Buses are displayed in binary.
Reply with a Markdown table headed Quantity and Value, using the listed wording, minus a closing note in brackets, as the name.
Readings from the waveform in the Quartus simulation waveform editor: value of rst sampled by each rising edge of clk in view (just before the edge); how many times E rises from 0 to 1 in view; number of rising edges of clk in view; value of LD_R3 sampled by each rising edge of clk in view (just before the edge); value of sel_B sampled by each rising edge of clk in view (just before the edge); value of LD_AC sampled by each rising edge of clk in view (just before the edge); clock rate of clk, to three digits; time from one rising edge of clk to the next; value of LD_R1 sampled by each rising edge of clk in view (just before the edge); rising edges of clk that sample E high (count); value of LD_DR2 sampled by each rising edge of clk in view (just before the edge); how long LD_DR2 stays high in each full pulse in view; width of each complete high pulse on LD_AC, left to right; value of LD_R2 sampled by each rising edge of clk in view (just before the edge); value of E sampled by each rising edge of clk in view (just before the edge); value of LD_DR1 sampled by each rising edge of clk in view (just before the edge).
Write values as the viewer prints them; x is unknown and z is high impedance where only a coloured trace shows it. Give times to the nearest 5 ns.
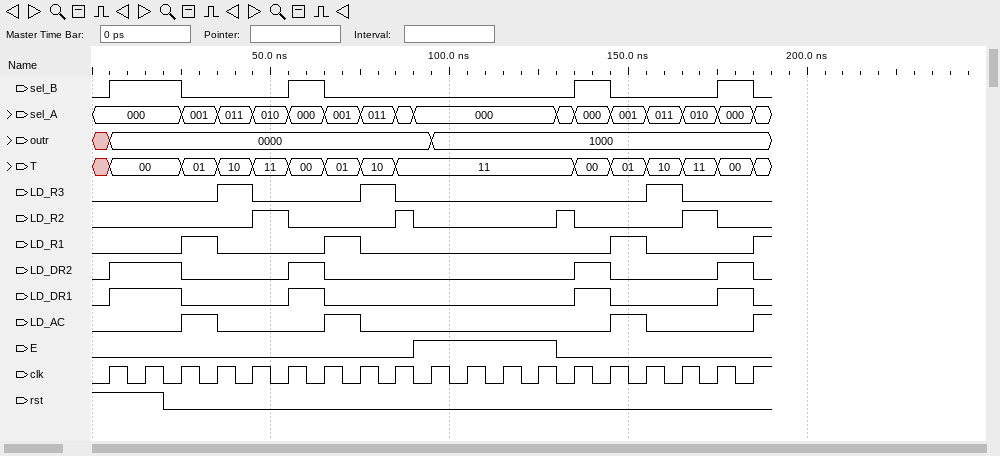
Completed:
| Quantity | Value |
|---|---|
| value of rst sampled by each rising edge of clk in view | 1 1 0 0 0 0 0 0 0 0 0 0 0 0 0 0 0 0 0 |
| how many times E rises from 0 to 1 in view | 1 |
| number of rising edges of clk in view | 19 |
| value of LD_R3 sampled by each rising edge of clk in view | 0 0 0 0 1 0 0 0 1 0 0 0 0 0 0 0 1 0 0 |
| value of sel_B sampled by each rising edge of clk in view | 0 1 1 0 0 0 1 0 0 0 0 0 0 0 1 0 0 0 1 |
| value of LD_AC sampled by each rising edge of clk in view | 0 0 0 1 0 0 0 1 0 0 0 0 0 0 0 1 0 0 0 |
| clock rate of clk, to three digits | 100 MHz |
| time from one rising edge of clk to the next | 10 ns |
| value of LD_R1 sampled by each rising edge of clk in view | 0 0 0 1 0 0 0 1 0 0 0 0 0 0 0 1 0 0 0 |
| rising edges of clk that sample E high | 4 |
| value of LD_DR2 sampled by each rising edge of clk in view | 0 1 1 0 0 0 1 0 0 0 0 0 0 0 1 0 0 0 1 |
| how long LD_DR2 stays high in each full pulse in view | 20 ns, 10 ns, 10 ns, 10 ns |
| width of each complete high pulse on LD_AC, left to right | 10 ns, 10 ns, 10 ns |
| value of LD_R2 sampled by each rising edge of clk in view | 0 0 0 0 0 1 0 0 0 0 0 0 0 1 0 0 0 1 0 |
| value of E sampled by each rising edge of clk in view | 0 0 0 0 0 0 0 0 0 1 1 1 1 0 0 0 0 0 0 |
| value of LD_DR1 sampled by each rising edge of clk in view | 0 1 1 0 0 0 1 0 0 0 0 0 0 0 1 0 0 0 1 |
